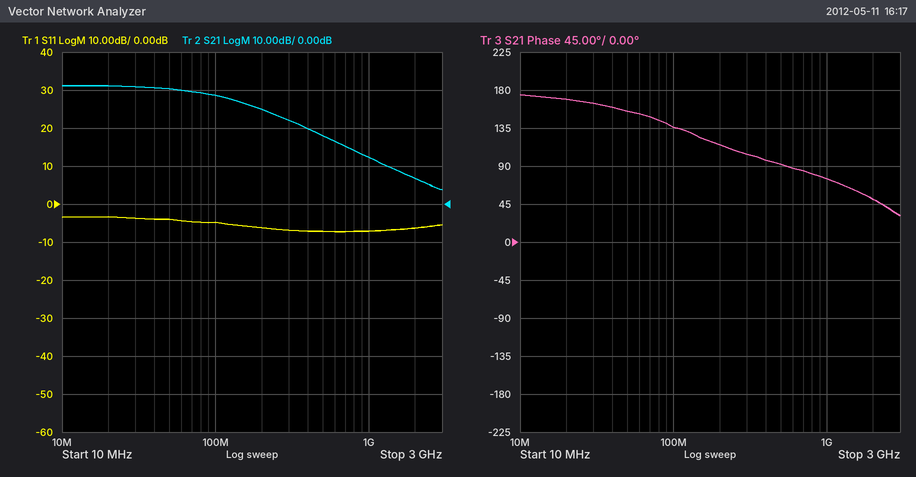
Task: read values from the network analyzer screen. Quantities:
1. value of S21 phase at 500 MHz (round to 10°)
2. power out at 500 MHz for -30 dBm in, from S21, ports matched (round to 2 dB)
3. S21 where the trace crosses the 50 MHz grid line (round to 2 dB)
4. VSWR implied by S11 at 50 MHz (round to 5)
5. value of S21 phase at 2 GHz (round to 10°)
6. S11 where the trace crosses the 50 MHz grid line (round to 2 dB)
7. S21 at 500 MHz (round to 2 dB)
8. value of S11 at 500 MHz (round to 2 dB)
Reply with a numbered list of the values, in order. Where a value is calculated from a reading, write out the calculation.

1. 90°
2. -30 dBm + (18 dB) = -12 dBm
3. 30 dB
4. |Γ| = 10^(-4/20) = 0.6310; VSWR = (1 + 0.6310)/(1 − 0.6310) ≈ 4.42, so 5 to the nearest 5
5. 50°
6. -4 dB
7. 18 dB
8. -8 dB
